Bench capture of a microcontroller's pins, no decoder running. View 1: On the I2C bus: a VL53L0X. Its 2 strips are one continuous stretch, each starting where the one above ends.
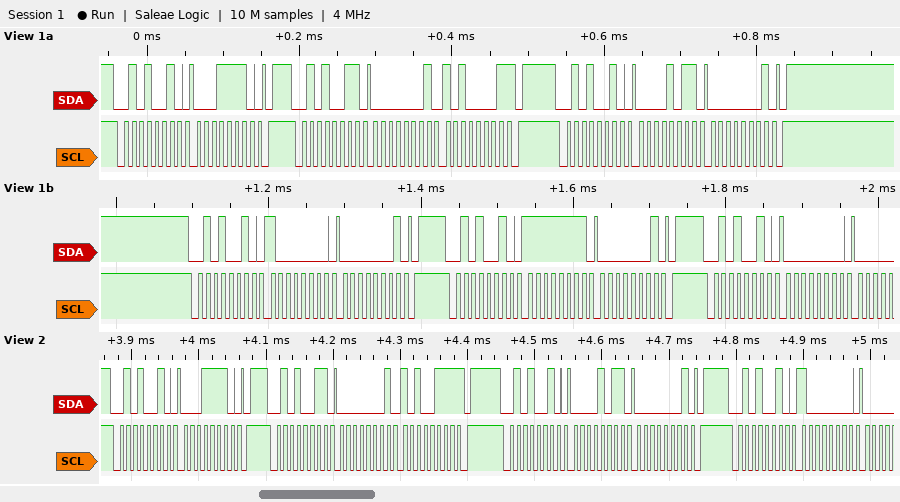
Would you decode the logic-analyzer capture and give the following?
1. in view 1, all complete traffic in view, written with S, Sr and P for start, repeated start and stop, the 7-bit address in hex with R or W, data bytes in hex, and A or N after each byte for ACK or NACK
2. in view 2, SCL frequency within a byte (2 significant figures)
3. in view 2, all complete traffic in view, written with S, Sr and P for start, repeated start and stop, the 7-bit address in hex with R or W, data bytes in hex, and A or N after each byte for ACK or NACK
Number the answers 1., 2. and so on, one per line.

1. S 29W A 1E A P S 29R A 01 A A1 N P S 29W A 0B A 01 A P S 29W A 80 A 01 A P S 29W A FF A 01 A P S 29W A 00 A
2. 100 kHz
3. S 29W A 1E A P S 29R A 01 A A7 N P S 29W A 0B A 01 A P S 29W A 80 A
